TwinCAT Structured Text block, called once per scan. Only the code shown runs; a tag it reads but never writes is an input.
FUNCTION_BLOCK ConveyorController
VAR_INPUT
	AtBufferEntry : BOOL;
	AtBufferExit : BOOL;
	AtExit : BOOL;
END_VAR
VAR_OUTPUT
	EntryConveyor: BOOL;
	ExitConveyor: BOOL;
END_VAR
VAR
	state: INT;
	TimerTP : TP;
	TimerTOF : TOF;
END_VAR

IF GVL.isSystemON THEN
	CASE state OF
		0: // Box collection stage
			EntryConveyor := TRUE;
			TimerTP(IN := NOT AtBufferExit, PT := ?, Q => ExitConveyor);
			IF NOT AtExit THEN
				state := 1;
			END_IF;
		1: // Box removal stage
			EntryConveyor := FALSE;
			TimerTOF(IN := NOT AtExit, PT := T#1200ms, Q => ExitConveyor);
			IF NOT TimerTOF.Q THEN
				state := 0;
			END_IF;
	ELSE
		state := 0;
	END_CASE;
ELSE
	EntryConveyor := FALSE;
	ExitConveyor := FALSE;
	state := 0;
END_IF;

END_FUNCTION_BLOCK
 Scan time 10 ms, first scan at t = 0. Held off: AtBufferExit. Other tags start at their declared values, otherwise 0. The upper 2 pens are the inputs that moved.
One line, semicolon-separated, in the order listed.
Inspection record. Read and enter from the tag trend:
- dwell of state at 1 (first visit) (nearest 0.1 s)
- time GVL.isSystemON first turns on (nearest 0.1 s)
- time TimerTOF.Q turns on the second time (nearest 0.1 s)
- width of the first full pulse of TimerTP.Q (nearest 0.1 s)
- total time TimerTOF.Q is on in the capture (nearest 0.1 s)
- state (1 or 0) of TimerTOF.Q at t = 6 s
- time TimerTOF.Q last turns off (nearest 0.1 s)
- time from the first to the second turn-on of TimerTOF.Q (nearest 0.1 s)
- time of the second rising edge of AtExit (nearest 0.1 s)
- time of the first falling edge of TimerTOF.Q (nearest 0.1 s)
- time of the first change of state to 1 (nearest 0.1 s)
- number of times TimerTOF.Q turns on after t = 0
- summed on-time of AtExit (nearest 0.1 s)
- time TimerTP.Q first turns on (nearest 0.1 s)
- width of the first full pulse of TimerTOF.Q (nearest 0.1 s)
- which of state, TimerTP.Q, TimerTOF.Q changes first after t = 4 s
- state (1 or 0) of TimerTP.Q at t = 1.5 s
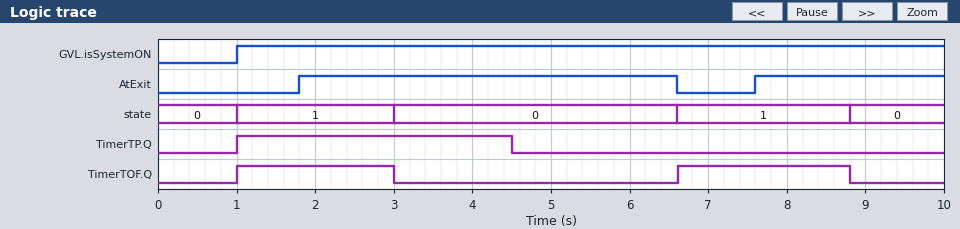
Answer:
2.0 s; 1.0 s; 6.6 s; 3.5 s; 4.2 s; 0; 8.8 s; 5.6 s; 7.6 s; 3.0 s; 1.0 s; 2; 7.2 s; 1.0 s; 2.0 s; TimerTP.Q; 1
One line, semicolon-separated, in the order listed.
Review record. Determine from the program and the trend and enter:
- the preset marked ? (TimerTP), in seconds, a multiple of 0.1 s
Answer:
3.5 s
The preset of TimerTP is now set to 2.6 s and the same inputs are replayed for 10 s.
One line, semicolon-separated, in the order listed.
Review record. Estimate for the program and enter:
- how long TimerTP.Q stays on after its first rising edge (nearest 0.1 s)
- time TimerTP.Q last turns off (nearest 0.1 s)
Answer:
2.6 s; 3.6 s
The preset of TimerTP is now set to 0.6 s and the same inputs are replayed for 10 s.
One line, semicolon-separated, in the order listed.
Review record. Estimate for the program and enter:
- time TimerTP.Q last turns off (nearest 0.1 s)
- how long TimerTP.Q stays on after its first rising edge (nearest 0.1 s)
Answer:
3.0 s; 2.0 s
